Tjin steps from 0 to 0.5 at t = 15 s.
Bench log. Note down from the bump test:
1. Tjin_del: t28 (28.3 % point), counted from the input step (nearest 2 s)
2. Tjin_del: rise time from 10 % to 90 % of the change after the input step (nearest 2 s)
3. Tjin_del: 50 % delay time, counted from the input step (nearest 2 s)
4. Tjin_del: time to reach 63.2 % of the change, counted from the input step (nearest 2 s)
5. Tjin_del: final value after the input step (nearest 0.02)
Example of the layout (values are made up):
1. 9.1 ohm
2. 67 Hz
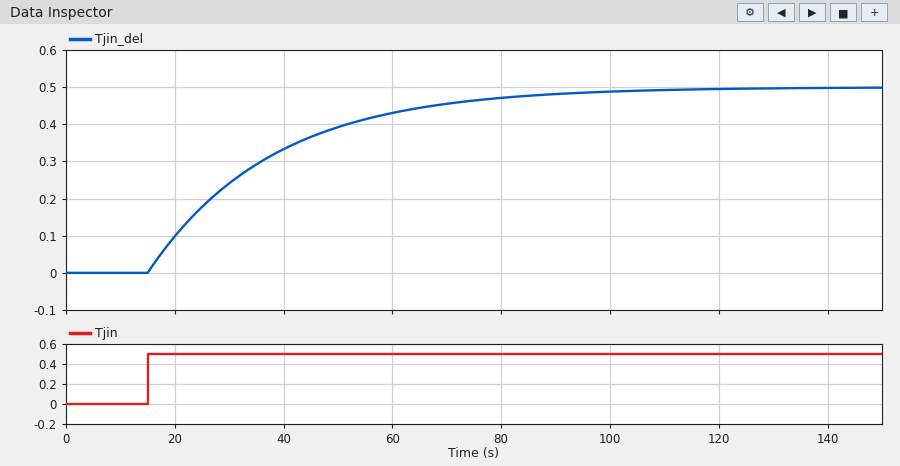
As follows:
1. 8 s
2. 50 s
3. 16 s
4. 22 s
5. 0.50
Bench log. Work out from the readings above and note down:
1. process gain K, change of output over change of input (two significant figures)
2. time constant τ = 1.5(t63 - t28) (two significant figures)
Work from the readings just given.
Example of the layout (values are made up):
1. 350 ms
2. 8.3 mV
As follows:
1. 1.0
2. 21 s
